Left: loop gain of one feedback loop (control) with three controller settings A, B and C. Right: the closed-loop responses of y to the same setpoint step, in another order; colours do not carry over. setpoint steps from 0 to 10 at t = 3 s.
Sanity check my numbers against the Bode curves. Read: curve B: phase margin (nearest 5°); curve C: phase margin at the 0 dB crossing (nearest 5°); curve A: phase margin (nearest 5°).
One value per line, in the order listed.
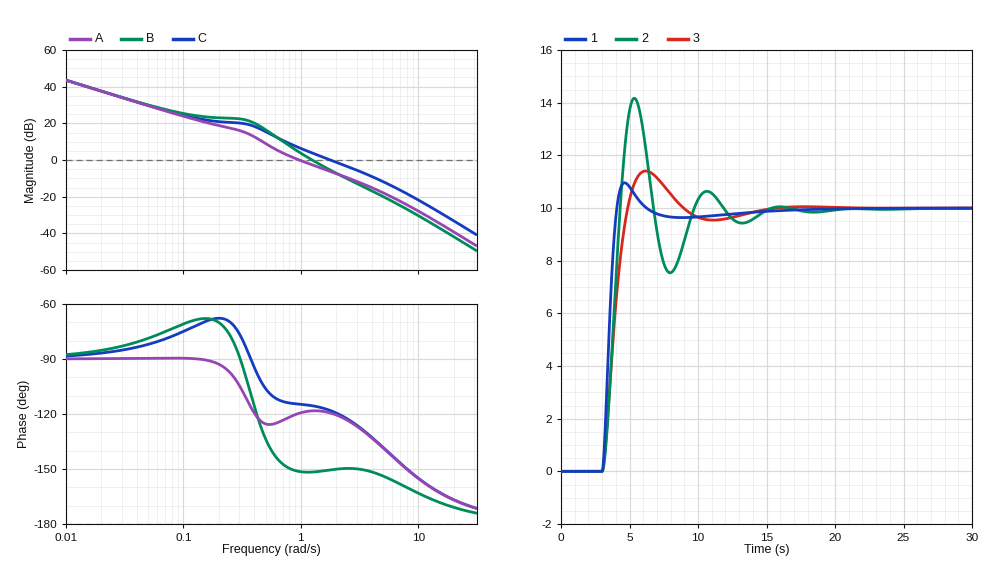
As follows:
30°
60°
60°
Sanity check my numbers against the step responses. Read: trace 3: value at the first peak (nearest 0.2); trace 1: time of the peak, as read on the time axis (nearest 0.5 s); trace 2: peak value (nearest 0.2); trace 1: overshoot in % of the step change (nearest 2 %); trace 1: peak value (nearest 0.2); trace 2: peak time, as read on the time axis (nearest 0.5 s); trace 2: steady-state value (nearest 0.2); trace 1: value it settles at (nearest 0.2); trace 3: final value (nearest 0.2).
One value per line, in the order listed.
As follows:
11.4
4.5 s
14.2
10 %
11.0
5.5 s
10.0
10.0
10.0
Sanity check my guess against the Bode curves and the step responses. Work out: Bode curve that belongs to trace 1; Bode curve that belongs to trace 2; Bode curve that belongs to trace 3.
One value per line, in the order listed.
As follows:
C
B
A
